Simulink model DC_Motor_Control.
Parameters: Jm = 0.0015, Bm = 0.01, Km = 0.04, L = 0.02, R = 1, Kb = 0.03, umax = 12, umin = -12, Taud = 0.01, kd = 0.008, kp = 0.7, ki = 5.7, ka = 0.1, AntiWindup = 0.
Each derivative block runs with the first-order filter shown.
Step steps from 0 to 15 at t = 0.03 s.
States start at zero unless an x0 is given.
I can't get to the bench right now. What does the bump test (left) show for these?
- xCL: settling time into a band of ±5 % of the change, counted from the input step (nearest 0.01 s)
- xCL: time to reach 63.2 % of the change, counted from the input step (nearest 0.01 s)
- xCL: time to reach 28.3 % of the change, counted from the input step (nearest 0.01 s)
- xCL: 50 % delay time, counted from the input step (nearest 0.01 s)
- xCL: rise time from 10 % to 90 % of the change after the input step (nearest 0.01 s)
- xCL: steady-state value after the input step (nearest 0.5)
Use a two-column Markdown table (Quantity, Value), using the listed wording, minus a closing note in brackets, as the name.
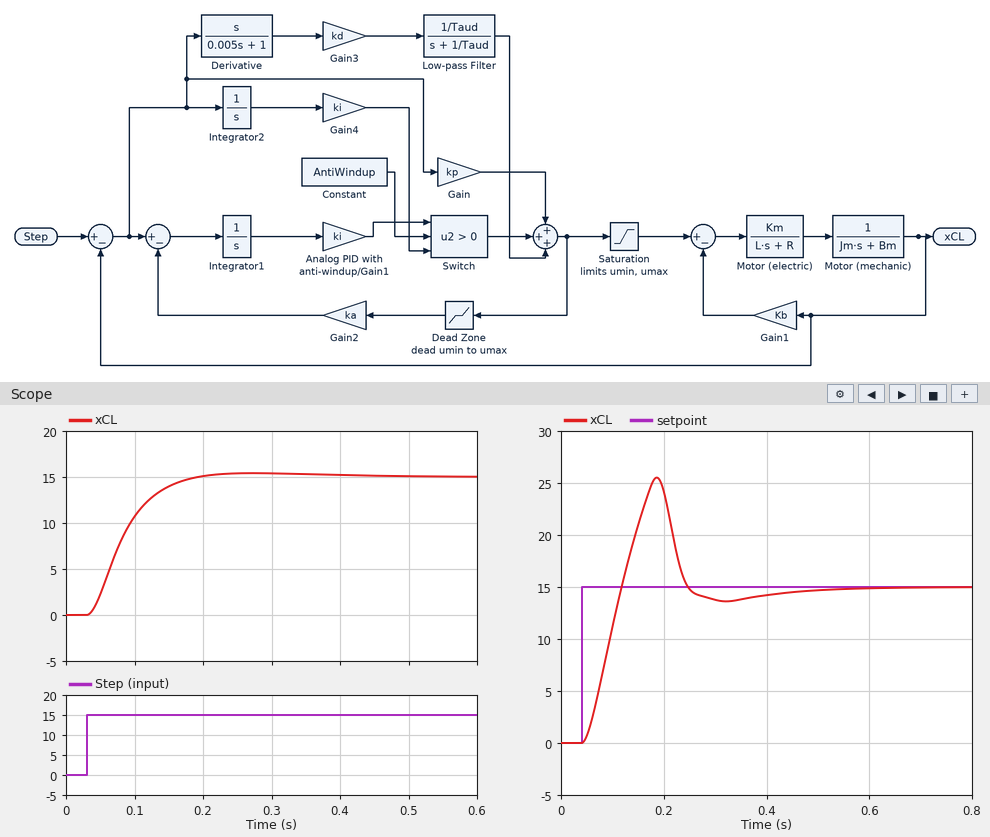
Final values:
| Quantity | Value |
|---|---|
| xCL: settling time into a band of ±5 % of the change, counted from the input step | 0.13 s |
| xCL: time to reach 63.2 % of the change, counted from the input step | 0.06 s |
| xCL: time to reach 28.3 % of the change, counted from the input step | 0.03 s |
| xCL: 50 % delay time, counted from the input step | 0.05 s |
| xCL: rise time from 10 % to 90 % of the change after the input step | 0.09 s |
| xCL: steady-state value after the input step | 15.0 |
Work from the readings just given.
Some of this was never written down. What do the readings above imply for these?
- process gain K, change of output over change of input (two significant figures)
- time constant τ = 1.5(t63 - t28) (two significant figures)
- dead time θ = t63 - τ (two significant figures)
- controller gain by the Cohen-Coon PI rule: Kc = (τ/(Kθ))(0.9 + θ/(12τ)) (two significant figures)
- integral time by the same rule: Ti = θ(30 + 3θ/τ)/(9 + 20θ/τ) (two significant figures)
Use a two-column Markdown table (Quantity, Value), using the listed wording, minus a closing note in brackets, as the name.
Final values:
| Quantity | Value |
|---|---|
| process gain K, change of output over change of input | 1.0 |
| time constant τ = 1.5(t63 - t28) | 0.045 s |
| dead time θ = t63 - τ | 0.015 s |
| controller gain by the Cohen-Coon PI rule: Kc = (τ/(Kθ))(0.9 + θ/(12τ)) | 2.8 |
| integral time by the same rule: Ti = θ(30 + 3θ/τ)/(9 + 20θ/τ) | 0.030 s |
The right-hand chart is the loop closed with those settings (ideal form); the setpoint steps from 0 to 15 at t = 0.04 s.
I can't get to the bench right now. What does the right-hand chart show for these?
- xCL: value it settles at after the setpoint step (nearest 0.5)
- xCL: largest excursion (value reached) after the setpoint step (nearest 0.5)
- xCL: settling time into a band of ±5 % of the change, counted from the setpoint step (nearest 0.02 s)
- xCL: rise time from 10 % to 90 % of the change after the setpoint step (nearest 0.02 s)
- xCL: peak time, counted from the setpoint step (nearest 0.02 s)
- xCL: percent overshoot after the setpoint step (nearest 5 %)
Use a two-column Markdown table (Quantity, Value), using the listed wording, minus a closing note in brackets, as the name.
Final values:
| Quantity | Value |
|---|---|
| xCL: value it settles at after the setpoint step | 15.0 |
| xCL: largest excursion (value reached) after the setpoint step | 25.5 |
| xCL: settling time into a band of ±5 % of the change, counted from the setpoint step | 0.36 s |
| xCL: rise time from 10 % to 90 % of the change after the setpoint step | 0.06 s |
| xCL: peak time, counted from the setpoint step | 0.14 s |
| xCL: percent overshoot after the setpoint step | 70 % |
